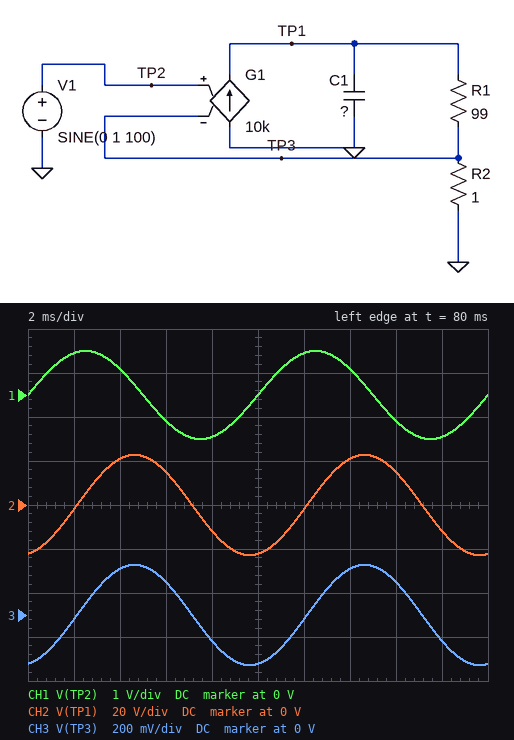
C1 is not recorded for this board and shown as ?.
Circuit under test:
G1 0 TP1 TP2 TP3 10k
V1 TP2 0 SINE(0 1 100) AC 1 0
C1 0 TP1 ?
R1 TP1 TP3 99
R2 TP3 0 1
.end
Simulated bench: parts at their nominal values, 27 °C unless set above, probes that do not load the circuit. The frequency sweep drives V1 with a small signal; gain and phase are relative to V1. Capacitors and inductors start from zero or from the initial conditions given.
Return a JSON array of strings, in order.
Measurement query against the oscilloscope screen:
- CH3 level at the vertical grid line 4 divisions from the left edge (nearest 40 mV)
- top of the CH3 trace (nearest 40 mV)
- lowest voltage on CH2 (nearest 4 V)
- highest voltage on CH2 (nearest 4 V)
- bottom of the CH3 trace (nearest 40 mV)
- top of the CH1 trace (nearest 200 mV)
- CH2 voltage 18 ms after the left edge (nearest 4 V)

["-120 mV", "240 mV", "-24 V", "24 V", "-240 mV", "1.0 V", "-12 V"]
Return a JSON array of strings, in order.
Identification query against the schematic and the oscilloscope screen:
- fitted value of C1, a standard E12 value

["680 mF"]
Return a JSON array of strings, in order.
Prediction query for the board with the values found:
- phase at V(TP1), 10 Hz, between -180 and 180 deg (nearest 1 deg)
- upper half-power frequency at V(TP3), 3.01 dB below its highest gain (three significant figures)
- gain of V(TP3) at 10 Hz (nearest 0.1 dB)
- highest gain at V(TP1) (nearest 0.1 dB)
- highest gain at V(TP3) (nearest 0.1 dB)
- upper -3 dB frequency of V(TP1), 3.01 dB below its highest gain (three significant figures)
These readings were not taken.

["-23 deg", "23.4 Hz", "-0.7 dB", "40.0 dB", "0 dB", "23.4 Hz"]
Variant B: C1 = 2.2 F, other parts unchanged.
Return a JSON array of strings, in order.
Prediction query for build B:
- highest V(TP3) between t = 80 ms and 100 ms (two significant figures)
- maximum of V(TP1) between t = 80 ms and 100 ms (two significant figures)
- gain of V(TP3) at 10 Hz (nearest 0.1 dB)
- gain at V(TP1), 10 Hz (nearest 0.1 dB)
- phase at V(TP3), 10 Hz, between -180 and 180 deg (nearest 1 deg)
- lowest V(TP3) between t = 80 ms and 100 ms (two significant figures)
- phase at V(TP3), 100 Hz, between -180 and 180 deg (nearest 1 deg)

["74 mV", "7.4 V", "-4.6 dB", "35.4 dB", "-54 deg", "-71 mV", "-86 deg"]
